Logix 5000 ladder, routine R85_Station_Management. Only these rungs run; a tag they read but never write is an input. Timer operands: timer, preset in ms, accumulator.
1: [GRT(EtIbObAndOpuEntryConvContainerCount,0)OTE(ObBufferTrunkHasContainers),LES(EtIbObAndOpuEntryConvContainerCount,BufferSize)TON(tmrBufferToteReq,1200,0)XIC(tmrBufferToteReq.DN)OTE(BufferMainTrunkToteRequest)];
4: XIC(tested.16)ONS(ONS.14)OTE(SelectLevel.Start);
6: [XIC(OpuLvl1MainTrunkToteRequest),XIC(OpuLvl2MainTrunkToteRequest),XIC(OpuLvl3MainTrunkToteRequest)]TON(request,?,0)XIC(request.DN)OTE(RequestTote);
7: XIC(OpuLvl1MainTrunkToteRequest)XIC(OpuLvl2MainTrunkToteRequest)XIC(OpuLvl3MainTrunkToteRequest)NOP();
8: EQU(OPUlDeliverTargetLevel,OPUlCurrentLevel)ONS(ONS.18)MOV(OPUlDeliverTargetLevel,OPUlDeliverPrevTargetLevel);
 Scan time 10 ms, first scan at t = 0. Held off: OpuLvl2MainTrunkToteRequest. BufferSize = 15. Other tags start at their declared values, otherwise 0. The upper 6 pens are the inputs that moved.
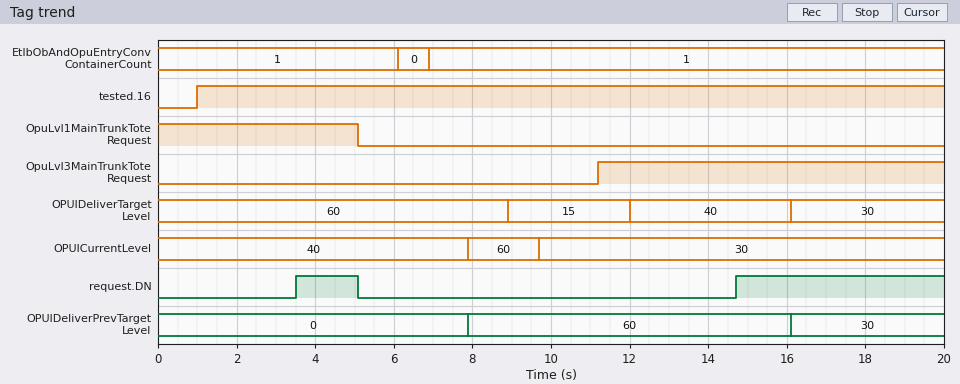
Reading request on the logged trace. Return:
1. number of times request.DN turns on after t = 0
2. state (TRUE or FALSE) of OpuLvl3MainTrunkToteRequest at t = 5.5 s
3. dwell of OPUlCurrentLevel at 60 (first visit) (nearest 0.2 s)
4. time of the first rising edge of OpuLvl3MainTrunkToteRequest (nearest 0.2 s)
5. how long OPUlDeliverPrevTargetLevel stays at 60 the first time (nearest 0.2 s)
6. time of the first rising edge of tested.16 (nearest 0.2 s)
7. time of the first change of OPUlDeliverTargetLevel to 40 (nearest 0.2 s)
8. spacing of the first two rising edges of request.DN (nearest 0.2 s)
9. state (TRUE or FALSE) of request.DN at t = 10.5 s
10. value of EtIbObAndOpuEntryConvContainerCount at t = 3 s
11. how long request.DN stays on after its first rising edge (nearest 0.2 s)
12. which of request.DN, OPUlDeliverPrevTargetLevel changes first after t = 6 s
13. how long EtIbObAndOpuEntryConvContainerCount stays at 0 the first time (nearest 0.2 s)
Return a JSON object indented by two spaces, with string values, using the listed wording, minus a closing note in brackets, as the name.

{
  "number of times request.DN turns on after t = 0": "2",
  "state (TRUE or FALSE) of OpuLvl3MainTrunkToteRequest at t = 5.5 s": "FALSE",
  "dwell of OPUlCurrentLevel at 60 (first visit)": "1.8 s",
  "time of the first rising edge of OpuLvl3MainTrunkToteRequest": "11.2 s",
  "how long OPUlDeliverPrevTargetLevel stays at 60 the first time": "8.2 s",
  "time of the first rising edge of tested.16": "1.0 s",
  "time of the first change of OPUlDeliverTargetLevel to 40": "12.0 s",
  "spacing of the first two rising edges of request.DN": "11.2 s",
  "state (TRUE or FALSE) of request.DN at t = 10.5 s": "FALSE",
  "value of EtIbObAndOpuEntryConvContainerCount at t = 3 s": "1",
  "how long request.DN stays on after its first rising edge": "1.6 s",
  "which of request.DN, OPUlDeliverPrevTargetLevel changes first after t = 6 s": "OPUlDeliverPrevTargetLevel",
  "how long EtIbObAndOpuEntryConvContainerCount stays at 0 the first time": "0.8 s"
}
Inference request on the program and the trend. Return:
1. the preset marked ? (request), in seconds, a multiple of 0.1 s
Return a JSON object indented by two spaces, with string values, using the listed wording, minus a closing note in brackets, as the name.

{
  "the preset marked ? (request), in seconds, a multiple of 0.1 s": "3.5 s"
}
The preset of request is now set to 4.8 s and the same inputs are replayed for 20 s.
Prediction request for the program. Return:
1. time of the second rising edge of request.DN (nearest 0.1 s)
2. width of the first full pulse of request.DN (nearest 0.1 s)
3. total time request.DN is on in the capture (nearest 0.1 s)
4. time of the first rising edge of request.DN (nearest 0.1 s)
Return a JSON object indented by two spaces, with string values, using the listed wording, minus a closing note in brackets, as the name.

{
  "time of the second rising edge of request.DN": "16.0 s",
  "width of the first full pulse of request.DN": "0.3 s",
  "total time request.DN is on in the capture": "4.3 s",
  "time of the first rising edge of request.DN": "4.8 s"
}
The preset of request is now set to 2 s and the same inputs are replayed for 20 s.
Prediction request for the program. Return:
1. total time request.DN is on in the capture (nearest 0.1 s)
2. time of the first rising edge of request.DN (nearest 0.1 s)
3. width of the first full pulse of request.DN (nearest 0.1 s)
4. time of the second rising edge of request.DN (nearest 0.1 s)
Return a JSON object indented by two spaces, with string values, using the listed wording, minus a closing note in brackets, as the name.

{
  "total time request.DN is on in the capture": "9.9 s",
  "time of the first rising edge of request.DN": "2.0 s",
  "width of the first full pulse of request.DN": "3.1 s",
  "time of the second rising edge of request.DN": "13.2 s"
}
